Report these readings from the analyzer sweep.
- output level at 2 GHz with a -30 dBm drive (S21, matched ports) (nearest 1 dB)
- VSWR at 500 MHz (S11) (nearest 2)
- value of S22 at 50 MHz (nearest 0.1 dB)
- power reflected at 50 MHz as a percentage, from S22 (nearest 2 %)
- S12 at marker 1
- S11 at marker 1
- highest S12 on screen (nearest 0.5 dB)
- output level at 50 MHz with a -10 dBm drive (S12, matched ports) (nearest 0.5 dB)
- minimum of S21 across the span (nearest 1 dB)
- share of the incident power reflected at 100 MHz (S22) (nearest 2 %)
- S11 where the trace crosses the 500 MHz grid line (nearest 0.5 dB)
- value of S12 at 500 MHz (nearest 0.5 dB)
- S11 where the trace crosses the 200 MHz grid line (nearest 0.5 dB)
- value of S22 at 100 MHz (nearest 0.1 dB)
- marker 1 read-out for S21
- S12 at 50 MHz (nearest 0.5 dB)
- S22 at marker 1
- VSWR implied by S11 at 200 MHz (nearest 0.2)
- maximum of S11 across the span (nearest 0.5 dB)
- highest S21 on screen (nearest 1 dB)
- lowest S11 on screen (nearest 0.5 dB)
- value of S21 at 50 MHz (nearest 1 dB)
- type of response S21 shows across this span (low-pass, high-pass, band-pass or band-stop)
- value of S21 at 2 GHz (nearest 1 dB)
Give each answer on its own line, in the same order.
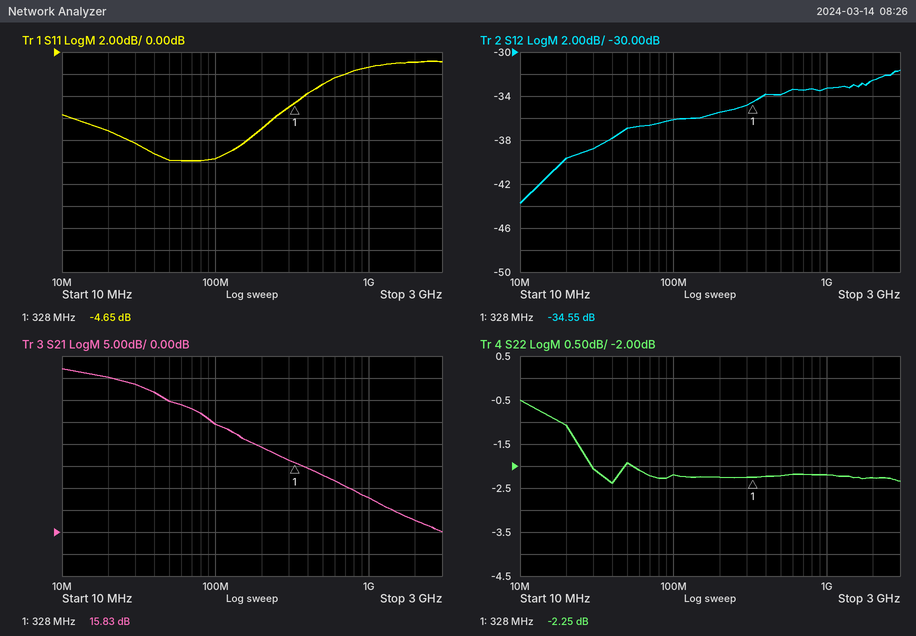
-27 dBm
6
-1.9 dB
64 %
-34.55 dB
-4.65 dB
-31.5 dB
-47.0 dBm
0 dB
60 %
-3.0 dB
-34.0 dB
-7.0 dB
-2.2 dB
15.83 dB
-37.0 dB
-2.25 dB
2.6
-1.0 dB
37 dB
-10.0 dB
30 dB
low-pass
3 dB
